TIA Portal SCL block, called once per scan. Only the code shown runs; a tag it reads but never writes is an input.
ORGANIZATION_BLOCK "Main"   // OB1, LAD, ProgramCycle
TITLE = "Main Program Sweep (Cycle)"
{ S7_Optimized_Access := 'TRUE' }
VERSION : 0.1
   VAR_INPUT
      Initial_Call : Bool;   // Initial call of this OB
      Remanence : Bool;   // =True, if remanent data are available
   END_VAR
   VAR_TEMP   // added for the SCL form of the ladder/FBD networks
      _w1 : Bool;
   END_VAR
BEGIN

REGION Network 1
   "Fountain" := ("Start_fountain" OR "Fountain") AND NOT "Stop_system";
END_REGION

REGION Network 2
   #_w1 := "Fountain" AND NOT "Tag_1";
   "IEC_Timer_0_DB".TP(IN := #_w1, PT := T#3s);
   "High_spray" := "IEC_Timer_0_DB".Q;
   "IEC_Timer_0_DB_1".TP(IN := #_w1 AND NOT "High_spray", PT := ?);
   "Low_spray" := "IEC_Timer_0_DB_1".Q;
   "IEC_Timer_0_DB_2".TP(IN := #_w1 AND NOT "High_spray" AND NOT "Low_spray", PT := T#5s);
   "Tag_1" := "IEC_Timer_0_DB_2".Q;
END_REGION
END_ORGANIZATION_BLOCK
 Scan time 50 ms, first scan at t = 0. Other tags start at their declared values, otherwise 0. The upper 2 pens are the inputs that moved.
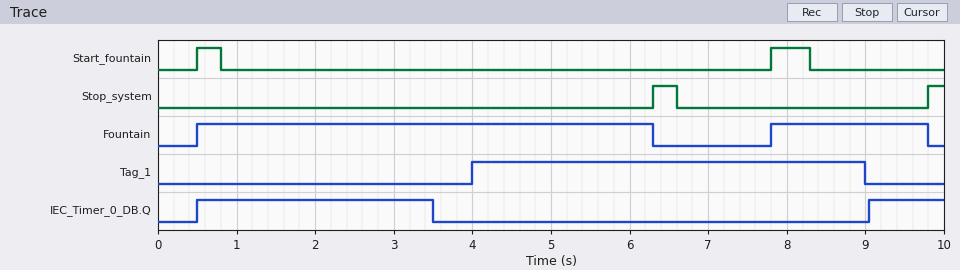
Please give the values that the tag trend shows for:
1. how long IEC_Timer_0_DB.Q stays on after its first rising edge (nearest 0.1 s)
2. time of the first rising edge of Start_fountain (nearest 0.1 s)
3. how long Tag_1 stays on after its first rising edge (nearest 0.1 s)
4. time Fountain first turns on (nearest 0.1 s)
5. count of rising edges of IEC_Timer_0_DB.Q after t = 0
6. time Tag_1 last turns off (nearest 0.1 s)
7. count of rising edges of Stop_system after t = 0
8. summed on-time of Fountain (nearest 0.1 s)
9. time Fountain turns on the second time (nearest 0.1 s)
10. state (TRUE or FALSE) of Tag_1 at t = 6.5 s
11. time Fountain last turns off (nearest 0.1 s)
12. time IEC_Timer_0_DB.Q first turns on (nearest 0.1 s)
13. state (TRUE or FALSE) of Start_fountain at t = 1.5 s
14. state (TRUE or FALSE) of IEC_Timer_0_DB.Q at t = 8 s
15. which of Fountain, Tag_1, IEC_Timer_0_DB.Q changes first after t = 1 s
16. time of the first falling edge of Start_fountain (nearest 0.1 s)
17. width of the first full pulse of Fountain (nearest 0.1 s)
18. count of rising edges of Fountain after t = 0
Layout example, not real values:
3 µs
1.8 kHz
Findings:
3.0 s
0.5 s
5.0 s
0.5 s
2
9.0 s
2
7.8 s
7.8 s
TRUE
9.8 s
0.5 s
FALSE
FALSE
IEC_Timer_0_DB.Q
0.8 s
5.8 s
2
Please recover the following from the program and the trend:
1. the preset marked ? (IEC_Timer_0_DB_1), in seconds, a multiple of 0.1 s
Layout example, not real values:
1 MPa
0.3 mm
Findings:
0.5 s
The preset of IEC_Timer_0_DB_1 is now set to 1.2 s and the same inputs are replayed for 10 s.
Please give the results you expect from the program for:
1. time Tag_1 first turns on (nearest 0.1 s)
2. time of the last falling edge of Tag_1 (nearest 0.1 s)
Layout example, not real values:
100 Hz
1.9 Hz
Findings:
4.7 s
9.7 s
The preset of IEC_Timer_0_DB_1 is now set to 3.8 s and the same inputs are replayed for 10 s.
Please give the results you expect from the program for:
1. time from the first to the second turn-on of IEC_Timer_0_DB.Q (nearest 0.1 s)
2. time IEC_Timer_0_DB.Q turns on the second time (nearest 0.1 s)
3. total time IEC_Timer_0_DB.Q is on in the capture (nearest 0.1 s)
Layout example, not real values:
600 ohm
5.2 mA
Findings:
7.3 s
7.8 s
5.2 s
